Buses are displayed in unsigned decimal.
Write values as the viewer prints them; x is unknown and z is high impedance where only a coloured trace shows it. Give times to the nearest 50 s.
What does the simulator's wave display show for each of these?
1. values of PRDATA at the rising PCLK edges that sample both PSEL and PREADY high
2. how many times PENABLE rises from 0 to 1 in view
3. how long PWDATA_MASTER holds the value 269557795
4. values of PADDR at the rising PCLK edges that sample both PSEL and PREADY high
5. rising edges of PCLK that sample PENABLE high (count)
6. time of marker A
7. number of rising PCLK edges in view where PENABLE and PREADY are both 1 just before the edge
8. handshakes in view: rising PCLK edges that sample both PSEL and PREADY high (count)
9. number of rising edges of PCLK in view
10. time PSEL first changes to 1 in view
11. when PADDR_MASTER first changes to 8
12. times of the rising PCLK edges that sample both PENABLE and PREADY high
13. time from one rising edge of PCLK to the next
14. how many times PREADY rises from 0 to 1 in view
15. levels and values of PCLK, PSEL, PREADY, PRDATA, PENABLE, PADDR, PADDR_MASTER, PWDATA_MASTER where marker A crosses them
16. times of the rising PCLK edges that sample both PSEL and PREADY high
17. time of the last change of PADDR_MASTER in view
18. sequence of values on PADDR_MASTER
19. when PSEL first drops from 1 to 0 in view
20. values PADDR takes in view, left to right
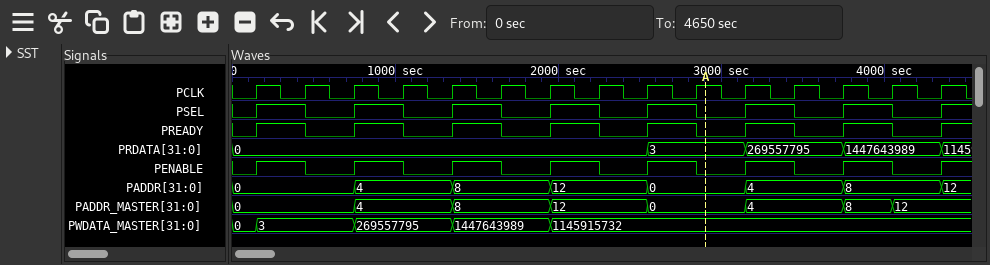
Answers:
0, 0, 0, 0, 3, 269557795, 1447643989
8
600 s
0, 4, 8, 12, 0, 4, 8
7
2900 s
7
7
15
150 s
1350 s
450 s, 1050 s, 1650 s, 2250 s, 2850 s, 3450 s, 4050 s
300 s
8
PCLK=1, PSEL=0, PREADY=0, PRDATA=3, PENABLE=0, PADDR=0, PADDR_MASTER=0, PWDATA_MASTER=1145915732
450 s, 1050 s, 1650 s, 2250 s, 2850 s, 3450 s, 4050 s
4050 s
0, 4, 8, 12, 0, 4, 8, 12
450 s
0, 4, 8, 12, 0, 4, 8, 12
